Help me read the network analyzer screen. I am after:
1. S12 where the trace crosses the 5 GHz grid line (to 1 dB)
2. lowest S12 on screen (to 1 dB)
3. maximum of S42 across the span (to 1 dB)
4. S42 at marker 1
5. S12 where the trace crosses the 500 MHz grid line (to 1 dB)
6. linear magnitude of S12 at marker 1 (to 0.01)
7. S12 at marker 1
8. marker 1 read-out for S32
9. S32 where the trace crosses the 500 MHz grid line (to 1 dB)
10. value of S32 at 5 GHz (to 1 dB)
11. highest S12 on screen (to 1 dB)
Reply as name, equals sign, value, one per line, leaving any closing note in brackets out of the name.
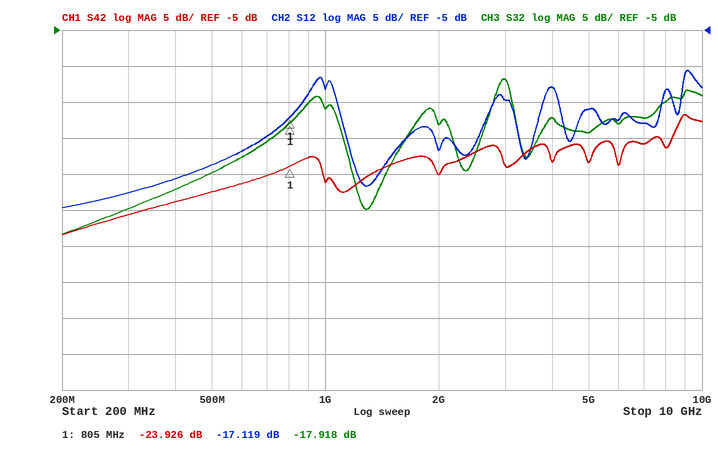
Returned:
S12 where the trace crosses the 5 GHz grid line = -16 dB
lowest S12 on screen = -30 dB
maximum of S42 across the span = -17 dB
S42 at marker 1 = -23.926 dB
S12 where the trace crosses the 500 MHz grid line = -24 dB
linear magnitude of S12 at marker 1 = 0.14
S12 at marker 1 = -17.119 dB
marker 1 read-out for S32 = -17.918 dB
S32 where the trace crosses the 500 MHz grid line = -25 dB
value of S32 at 5 GHz = -19 dB
highest S12 on screen = -11 dB
